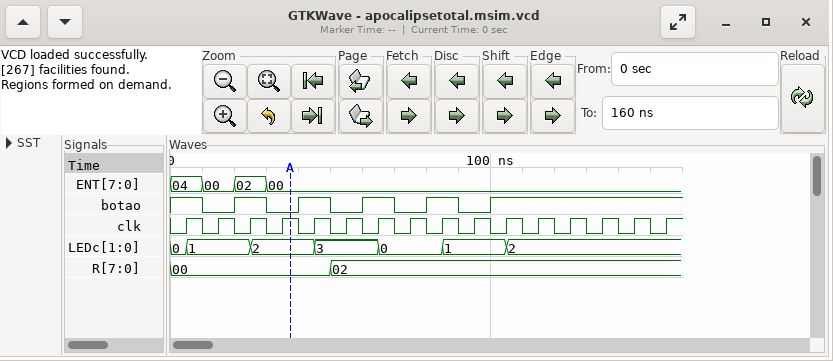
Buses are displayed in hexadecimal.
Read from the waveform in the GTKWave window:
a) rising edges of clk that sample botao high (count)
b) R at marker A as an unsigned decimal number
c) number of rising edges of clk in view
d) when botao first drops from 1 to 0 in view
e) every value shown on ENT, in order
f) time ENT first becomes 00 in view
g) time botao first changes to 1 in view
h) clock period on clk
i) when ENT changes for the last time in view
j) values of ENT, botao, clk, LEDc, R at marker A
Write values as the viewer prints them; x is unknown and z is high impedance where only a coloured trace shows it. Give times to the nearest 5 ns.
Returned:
11
0
16
10 ns
04, 00, 02, 00
10 ns
20 ns
10 ns
30 ns
ENT=00, botao=0, clk=1, LEDc=2, R=00
